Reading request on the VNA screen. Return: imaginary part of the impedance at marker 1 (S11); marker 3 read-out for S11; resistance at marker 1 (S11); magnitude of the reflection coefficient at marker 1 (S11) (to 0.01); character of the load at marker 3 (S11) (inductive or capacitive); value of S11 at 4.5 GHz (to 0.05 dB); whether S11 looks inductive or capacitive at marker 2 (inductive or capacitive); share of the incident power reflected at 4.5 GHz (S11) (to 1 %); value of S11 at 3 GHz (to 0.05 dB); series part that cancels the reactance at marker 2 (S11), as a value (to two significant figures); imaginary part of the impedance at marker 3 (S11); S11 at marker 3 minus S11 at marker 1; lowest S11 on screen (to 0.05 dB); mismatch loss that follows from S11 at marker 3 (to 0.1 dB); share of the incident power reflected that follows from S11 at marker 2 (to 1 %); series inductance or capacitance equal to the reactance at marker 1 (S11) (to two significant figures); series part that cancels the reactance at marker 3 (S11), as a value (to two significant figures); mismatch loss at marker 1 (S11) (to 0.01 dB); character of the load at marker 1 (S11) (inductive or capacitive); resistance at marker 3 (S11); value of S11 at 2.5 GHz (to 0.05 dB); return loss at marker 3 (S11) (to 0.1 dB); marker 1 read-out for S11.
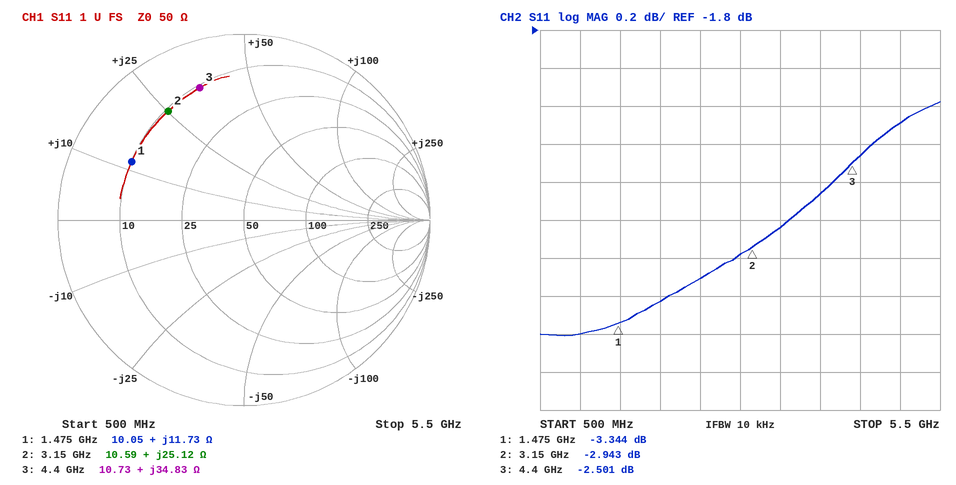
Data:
+11.73 Ω
-2.501 dB
10.05 Ω
0.68
inductive
-2.45 dB
inductive
57 %
-3.00 dB
2.0 pF
+34.83 Ω
0.843 dB
-3.40 dB
3.6 dB
51 %
1.3 nH
1.0 pF
2.70 dB
inductive
10.73 Ω
-3.10 dB
2.5 dB
-3.344 dB
